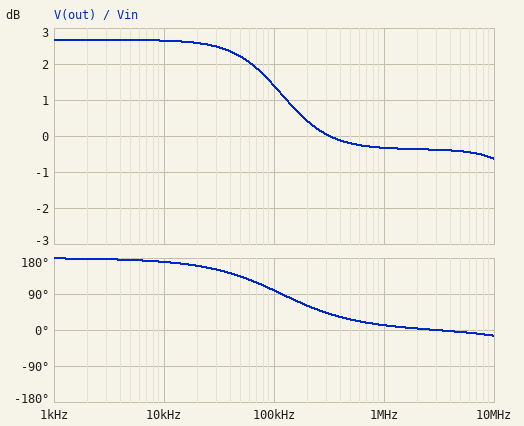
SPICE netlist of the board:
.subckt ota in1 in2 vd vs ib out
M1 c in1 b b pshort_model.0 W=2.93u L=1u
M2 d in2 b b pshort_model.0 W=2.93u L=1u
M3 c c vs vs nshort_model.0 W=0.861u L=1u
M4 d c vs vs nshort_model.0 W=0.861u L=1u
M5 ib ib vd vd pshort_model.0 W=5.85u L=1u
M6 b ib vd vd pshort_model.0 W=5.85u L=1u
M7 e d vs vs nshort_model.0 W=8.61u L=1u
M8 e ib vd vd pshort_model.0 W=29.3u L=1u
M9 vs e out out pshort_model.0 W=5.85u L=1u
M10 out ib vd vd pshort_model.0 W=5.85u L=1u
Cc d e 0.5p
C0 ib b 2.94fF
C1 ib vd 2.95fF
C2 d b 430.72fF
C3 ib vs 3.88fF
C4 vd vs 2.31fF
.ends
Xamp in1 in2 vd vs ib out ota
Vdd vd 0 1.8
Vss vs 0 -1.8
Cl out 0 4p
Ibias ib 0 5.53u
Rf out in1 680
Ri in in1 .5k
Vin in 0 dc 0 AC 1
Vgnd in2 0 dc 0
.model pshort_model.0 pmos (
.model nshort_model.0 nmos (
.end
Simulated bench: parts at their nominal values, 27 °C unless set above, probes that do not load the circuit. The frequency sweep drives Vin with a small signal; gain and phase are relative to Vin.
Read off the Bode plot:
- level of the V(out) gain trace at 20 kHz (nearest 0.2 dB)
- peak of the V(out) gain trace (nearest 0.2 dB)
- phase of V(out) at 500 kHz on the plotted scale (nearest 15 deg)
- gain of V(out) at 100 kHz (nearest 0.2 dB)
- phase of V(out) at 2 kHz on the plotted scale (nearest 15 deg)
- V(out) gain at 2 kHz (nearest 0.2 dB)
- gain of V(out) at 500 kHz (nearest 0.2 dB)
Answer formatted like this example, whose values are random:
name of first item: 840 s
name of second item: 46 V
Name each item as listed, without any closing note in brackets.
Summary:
level of the V(out) gain trace at 20 kHz: 2.6 dB
peak of the V(out) gain trace: 2.6 dB
phase of V(out) at 500 kHz on the plotted scale: 30 deg
gain of V(out) at 100 kHz: 1.4 dB
phase of V(out) at 2 kHz on the plotted scale: 180 deg
V(out) gain at 2 kHz: 2.6 dB
gain of V(out) at 500 kHz: -0.2 dB
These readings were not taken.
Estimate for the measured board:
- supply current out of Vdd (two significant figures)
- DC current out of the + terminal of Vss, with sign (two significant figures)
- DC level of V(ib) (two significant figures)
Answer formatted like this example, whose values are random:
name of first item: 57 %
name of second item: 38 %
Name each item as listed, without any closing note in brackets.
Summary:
supply current out of Vdd: 44 µA
DC current out of the + terminal of Vss, with sign: -39 µA
DC level of V(ib): 1.5 V
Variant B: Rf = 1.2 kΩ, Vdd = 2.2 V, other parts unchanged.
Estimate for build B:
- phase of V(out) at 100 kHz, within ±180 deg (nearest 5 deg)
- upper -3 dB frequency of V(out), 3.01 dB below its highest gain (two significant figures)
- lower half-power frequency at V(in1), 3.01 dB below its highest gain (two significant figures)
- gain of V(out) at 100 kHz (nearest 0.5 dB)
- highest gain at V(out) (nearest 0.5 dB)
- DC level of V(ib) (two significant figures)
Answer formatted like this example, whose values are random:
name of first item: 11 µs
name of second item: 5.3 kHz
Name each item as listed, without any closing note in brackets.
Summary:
phase of V(out) at 100 kHz, within ±180 deg: 110 deg
upper -3 dB frequency of V(out), 3.01 dB below its highest gain: 120 kHz
lower half-power frequency at V(in1), 3.01 dB below its highest gain: 97 kHz
gain of V(out) at 100 kHz: 5.0 dB
highest gain at V(out): 7.5 dB
DC level of V(ib): 1.9 V
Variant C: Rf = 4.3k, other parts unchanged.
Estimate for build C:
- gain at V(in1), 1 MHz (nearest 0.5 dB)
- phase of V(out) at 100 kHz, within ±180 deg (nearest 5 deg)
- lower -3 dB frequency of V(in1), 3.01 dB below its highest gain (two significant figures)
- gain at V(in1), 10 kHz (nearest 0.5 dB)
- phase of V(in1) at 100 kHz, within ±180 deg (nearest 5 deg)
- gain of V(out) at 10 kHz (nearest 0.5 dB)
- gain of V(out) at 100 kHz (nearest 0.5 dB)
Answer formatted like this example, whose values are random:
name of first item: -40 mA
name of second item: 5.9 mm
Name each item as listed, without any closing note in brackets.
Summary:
gain at V(in1), 1 MHz: 0 dB
phase of V(out) at 100 kHz, within ±180 deg: 125 deg
lower -3 dB frequency of V(in1), 3.01 dB below its highest gain: 88 kHz
gain at V(in1), 10 kHz: -19.0 dB
phase of V(in1) at 100 kHz, within ±180 deg: 40 deg
gain of V(out) at 10 kHz: 18.5 dB
gain of V(out) at 100 kHz: 15.0 dB
